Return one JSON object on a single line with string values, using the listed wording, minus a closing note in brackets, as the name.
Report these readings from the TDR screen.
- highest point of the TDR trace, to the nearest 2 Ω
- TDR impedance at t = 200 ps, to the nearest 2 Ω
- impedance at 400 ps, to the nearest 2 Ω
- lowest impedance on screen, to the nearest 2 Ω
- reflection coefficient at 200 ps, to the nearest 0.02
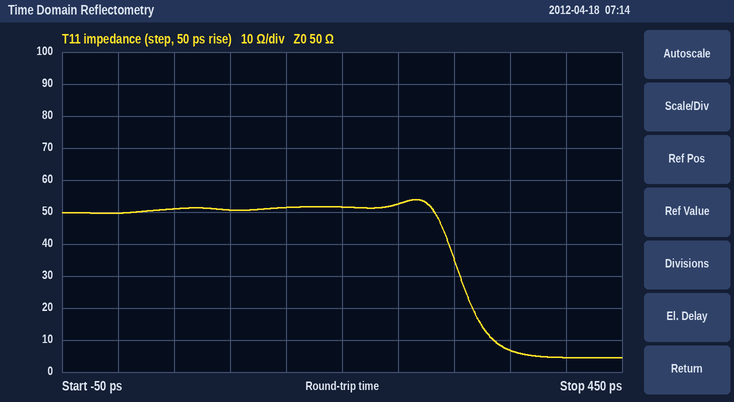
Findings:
{"highest point of the TDR trace, to the nearest 2 Ω": "54 Ω", "TDR impedance at t = 200 ps, to the nearest 2 Ω": "52 Ω", "impedance at 400 ps, to the nearest 2 Ω": "4 Ω", "lowest impedance on screen, to the nearest 2 Ω": "4 Ω", "reflection coefficient at 200 ps, to the nearest 0.02": "+0.02"}
